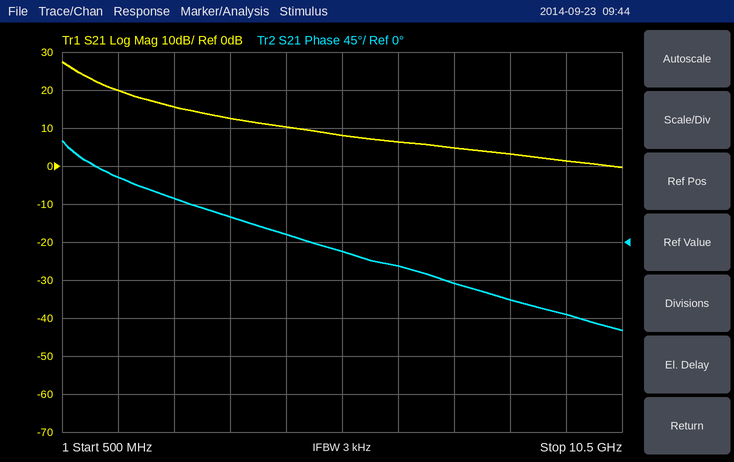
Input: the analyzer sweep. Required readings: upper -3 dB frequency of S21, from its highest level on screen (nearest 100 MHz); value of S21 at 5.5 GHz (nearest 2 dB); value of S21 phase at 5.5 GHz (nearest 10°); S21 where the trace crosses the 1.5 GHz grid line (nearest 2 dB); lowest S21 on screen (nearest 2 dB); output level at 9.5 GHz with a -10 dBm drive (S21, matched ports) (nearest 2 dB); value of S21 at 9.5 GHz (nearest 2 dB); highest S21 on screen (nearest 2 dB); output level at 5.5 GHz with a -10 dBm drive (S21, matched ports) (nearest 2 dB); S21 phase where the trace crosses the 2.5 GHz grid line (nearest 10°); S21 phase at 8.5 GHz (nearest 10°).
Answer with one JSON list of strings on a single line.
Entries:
["800 MHz", "8 dB", "-10°", "20 dB", "0 dB", "-8 dBm", "2 dB", "28 dB", "-2 dBm", "50°", "-70°"]
